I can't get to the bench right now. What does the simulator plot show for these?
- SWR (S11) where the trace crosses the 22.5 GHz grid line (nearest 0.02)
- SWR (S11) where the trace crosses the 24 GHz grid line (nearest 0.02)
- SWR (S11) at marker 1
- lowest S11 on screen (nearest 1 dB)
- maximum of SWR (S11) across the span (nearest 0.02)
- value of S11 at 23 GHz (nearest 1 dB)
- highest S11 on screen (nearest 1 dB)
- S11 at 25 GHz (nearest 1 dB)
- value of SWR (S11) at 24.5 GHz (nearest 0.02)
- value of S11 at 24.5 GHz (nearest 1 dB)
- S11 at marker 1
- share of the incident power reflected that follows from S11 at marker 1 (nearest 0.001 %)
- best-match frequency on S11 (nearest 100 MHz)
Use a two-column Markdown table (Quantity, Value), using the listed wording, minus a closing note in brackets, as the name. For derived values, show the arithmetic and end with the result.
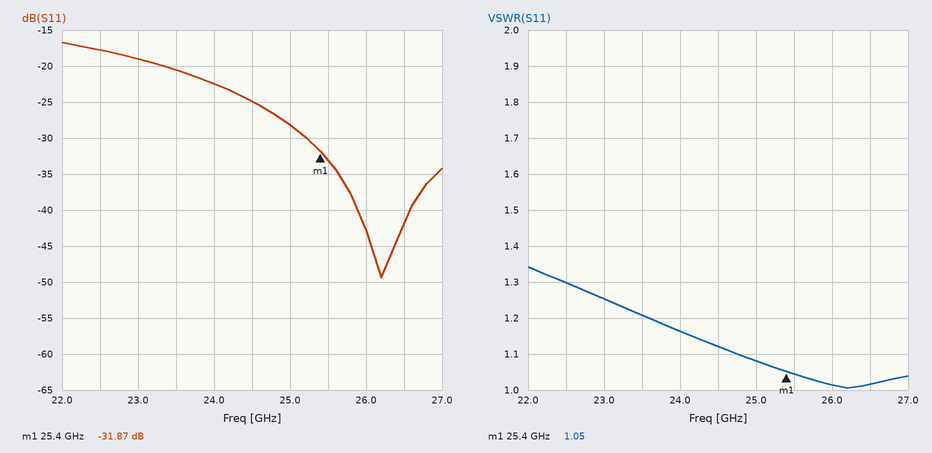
| Quantity | Value |
|---|---|
| SWR (S11) where the trace crosses the 22.5 GHz grid line | 1.30 |
| SWR (S11) where the trace crosses the 24 GHz grid line | 1.16 |
| SWR (S11) at marker 1 | 1.05 |
| lowest S11 on screen | -49 dB |
| maximum of SWR (S11) across the span | 1.34 |
| value of S11 at 23 GHz | -19 dB |
| highest S11 on screen | -17 dB |
| S11 at 25 GHz | -28 dB |
| value of SWR (S11) at 24.5 GHz | 1.12 |
| value of S11 at 24.5 GHz | -25 dB |
| S11 at marker 1 | -31.87 dB |
| share of the incident power reflected that follows from S11 at marker 1 | 10^(-31.87/10) ≈ 0.065 % |
| best-match frequency on S11 | 26.2 GHz |
